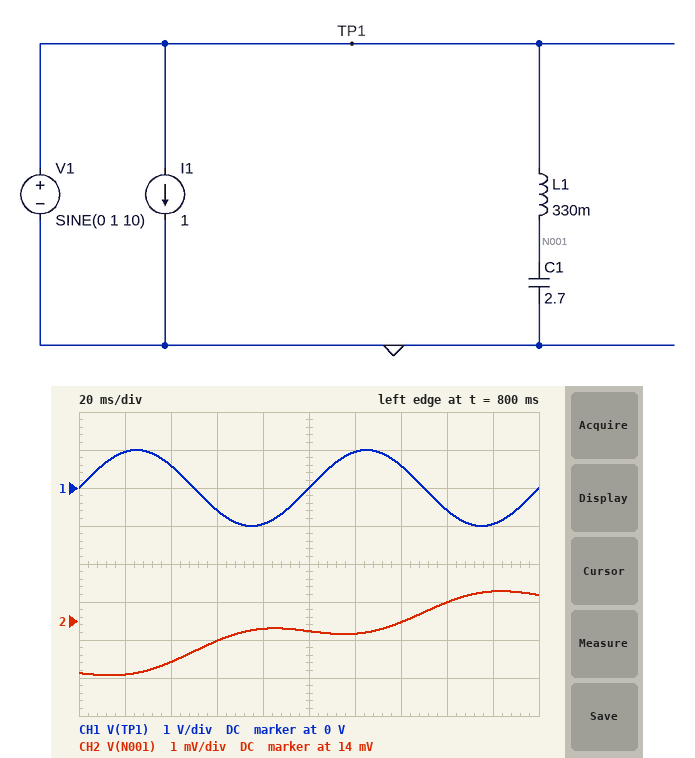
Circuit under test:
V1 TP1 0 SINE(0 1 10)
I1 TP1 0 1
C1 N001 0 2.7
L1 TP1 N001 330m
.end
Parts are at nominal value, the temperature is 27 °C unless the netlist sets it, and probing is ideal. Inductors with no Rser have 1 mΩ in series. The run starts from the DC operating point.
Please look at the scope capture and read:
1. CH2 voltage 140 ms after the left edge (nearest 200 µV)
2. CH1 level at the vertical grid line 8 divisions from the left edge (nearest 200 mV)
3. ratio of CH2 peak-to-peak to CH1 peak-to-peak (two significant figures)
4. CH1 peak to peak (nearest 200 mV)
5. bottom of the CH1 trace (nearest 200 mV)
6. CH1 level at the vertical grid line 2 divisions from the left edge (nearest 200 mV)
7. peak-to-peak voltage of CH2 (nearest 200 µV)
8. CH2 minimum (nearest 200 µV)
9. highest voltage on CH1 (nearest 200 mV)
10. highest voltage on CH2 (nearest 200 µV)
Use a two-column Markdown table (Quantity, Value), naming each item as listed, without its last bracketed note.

| Quantity | Value |
|---|---|
| CH2 voltage 140 ms after the left edge | 14.0 mV |
| CH1 level at the vertical grid line 8 divisions from the left edge | -600 mV |
| ratio of CH2 peak-to-peak to CH1 peak-to-peak | 0.0011 |
| CH1 peak to peak | 2.0 V |
| bottom of the CH1 trace | -1.0 V |
| CH1 level at the vertical grid line 2 divisions from the left edge | 600 mV |
| peak-to-peak voltage of CH2 | 2.2 mV |
| CH2 minimum | 12.6 mV |
| highest voltage on CH1 | 1.0 V |
| highest voltage on CH2 | 14.8 mV |
